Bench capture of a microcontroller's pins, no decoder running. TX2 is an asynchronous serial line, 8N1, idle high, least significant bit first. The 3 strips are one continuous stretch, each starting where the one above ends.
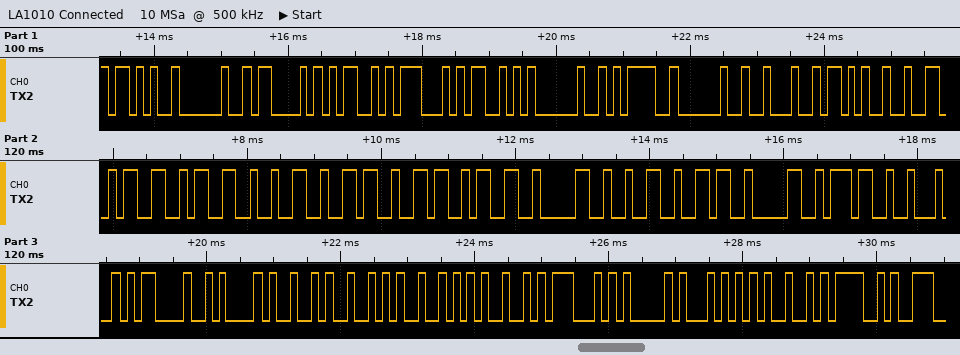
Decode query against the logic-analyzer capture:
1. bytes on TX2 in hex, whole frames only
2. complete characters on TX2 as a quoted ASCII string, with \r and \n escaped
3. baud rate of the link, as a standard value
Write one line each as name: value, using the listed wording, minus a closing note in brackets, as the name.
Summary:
bytes on TX2 in hex, whole frames only: 2B 20 43 4D 47 53 20 3D 20 22 2B 32 33 33 32 36 36 33 30 32 36 30 37 22 0D 0A 49 52 52 49 47 41 54 49 4F
complete characters on TX2 as a quoted ASCII string, with \r and \n escaped: "+ CMGS = \"+233266302607\"\r\nIRRIGATIO"
baud rate of the link, as a standard value: 9600 baud
